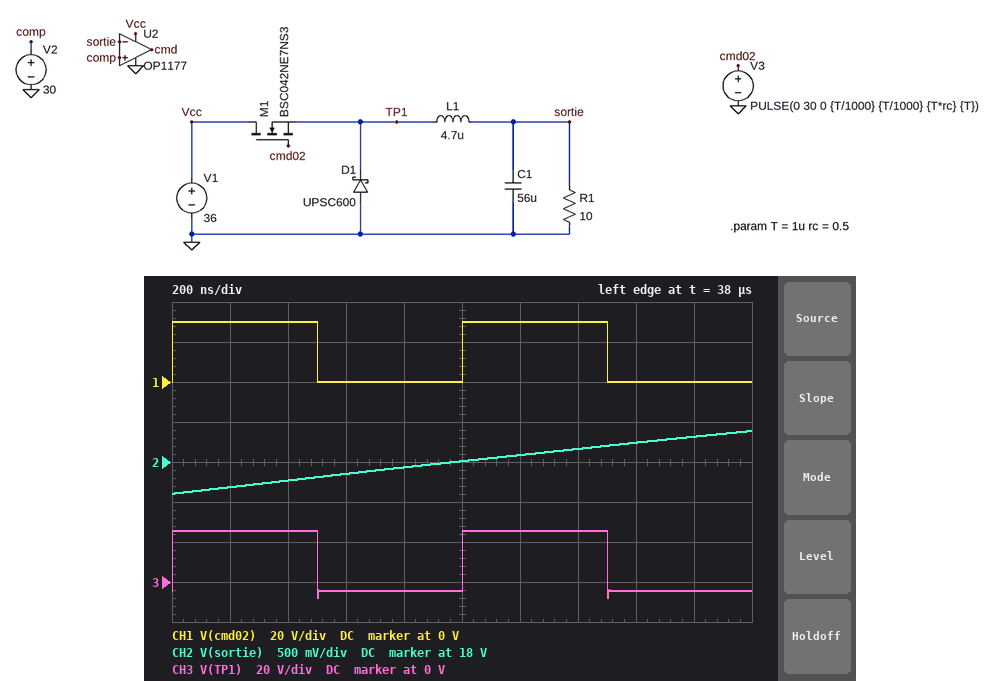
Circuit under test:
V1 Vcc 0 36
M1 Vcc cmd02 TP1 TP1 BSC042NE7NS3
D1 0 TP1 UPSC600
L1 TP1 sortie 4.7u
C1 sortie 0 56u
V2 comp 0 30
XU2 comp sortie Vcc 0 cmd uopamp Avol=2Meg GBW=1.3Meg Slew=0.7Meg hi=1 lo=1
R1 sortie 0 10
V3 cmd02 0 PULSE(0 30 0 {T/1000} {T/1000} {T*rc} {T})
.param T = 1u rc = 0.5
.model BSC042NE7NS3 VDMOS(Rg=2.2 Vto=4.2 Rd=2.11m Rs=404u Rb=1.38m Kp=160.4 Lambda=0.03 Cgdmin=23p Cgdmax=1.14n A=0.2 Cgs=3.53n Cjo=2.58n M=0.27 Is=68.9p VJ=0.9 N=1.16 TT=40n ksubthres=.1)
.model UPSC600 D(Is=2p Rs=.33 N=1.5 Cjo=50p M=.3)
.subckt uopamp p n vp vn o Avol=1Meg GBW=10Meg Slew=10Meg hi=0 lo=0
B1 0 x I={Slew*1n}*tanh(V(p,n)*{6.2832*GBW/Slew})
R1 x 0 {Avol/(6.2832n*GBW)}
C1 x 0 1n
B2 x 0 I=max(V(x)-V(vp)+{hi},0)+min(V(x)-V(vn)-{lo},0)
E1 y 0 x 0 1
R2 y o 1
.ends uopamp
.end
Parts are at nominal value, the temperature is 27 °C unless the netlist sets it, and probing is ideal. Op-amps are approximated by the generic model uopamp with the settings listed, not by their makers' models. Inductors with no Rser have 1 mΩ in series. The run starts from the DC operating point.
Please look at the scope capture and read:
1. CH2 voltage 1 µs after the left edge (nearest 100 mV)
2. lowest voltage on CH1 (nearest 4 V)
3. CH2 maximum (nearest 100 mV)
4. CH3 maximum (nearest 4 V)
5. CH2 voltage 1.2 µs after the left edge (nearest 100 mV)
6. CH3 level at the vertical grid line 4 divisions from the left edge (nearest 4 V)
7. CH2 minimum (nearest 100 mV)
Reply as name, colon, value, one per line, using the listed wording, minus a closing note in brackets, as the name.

CH2 voltage 1 µs after the left edge: 18.0 V
lowest voltage on CH1: 0 V
CH2 maximum: 18.4 V
CH3 maximum: 24 V
CH2 voltage 1.2 µs after the left edge: 18.1 V
CH3 level at the vertical grid line 4 divisions from the left edge: -4 V
CH2 minimum: 17.6 V
